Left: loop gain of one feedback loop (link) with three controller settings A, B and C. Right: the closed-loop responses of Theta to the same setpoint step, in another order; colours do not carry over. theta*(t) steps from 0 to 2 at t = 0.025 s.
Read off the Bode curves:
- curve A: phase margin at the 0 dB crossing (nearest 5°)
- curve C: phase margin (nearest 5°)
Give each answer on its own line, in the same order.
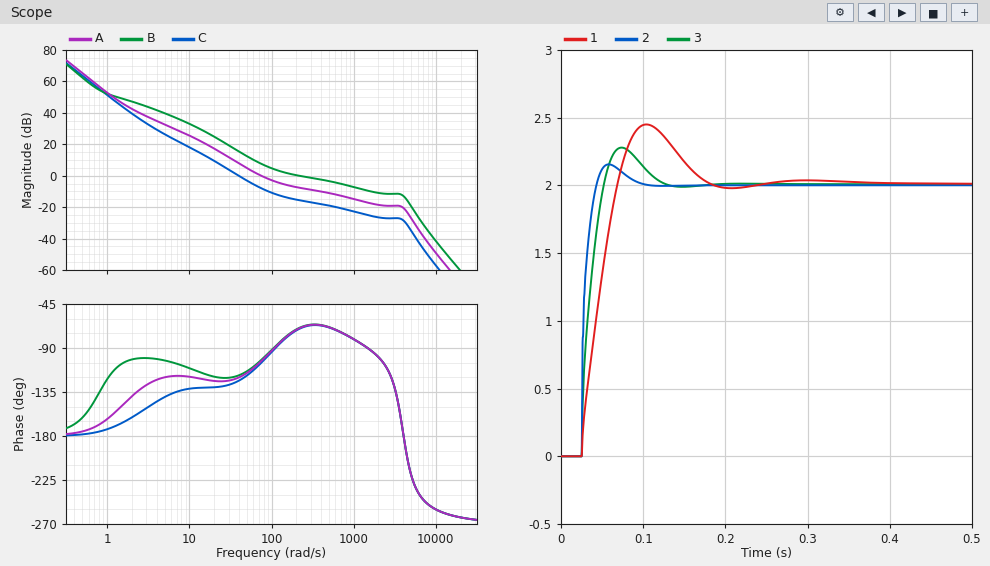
75°
55°
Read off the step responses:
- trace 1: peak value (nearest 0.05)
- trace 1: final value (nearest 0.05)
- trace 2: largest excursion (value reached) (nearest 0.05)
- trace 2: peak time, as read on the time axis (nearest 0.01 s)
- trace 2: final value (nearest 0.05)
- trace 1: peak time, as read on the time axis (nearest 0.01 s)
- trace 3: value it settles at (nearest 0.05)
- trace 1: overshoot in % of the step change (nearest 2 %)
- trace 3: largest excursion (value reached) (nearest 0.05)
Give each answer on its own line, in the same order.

2.45
2.00
2.15
0.06 s
2.00
0.10 s
2.00
22 %
2.30
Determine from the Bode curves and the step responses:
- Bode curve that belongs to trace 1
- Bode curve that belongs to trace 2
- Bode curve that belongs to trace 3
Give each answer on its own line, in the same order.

C
B
A
